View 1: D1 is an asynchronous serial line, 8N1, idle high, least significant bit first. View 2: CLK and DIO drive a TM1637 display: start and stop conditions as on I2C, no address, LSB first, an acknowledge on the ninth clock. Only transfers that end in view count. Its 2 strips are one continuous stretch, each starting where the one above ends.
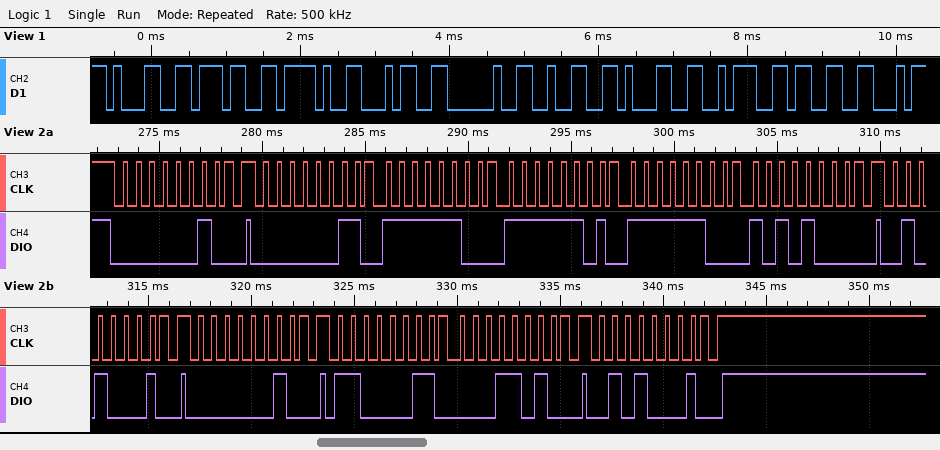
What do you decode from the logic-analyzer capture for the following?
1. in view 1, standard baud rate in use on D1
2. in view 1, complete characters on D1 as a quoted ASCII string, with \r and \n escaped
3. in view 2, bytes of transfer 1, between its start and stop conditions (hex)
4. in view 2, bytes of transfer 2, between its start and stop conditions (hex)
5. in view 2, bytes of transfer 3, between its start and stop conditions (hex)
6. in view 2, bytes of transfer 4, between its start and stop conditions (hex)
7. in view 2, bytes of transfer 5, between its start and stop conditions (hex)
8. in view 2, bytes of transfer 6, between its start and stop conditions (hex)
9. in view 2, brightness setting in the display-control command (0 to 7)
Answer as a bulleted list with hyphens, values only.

- 9600 baud
- "17/4 21:3"
- 40
- C0 3F BF 3F 15
- 8A
- 40
- C3 58
- 8A
- 2
